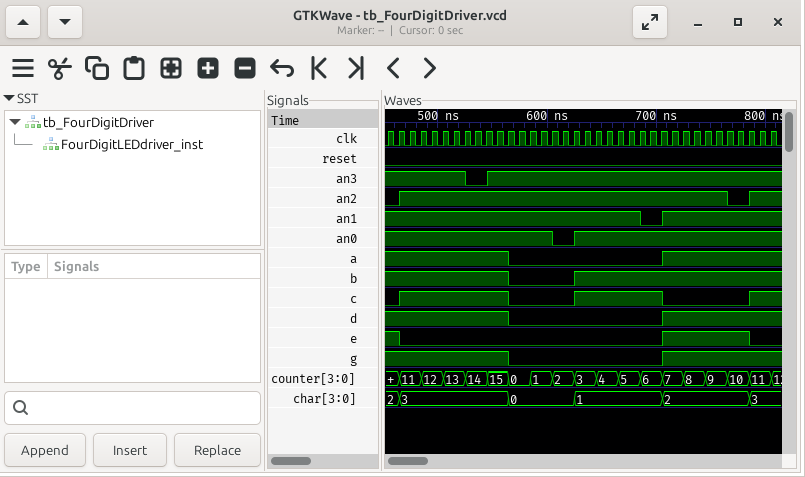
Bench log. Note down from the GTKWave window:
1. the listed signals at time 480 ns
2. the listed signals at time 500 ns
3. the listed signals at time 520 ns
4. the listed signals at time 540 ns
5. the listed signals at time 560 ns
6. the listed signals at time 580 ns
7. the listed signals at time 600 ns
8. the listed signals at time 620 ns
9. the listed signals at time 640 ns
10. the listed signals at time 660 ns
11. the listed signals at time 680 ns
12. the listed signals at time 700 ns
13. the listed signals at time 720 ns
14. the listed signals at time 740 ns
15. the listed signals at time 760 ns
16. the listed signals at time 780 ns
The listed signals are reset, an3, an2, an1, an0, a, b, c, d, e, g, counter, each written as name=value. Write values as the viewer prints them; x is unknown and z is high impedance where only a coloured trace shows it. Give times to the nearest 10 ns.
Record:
reset=0, an3=1, an2=1, an1=1, an0=1, a=1, b=1, c=1, d=1, e=0, g=1, counter=11
reset=0, an3=1, an2=1, an1=1, an0=1, a=1, b=1, c=1, d=1, e=0, g=1, counter=12
reset=0, an3=1, an2=1, an1=1, an0=1, a=1, b=1, c=1, d=1, e=0, g=1, counter=13
reset=0, an3=0, an2=1, an1=1, an0=1, a=1, b=1, c=1, d=1, e=0, g=1, counter=14
reset=0, an3=1, an2=1, an1=1, an0=1, a=1, b=1, c=1, d=1, e=0, g=1, counter=15
reset=0, an3=1, an2=1, an1=1, an0=1, a=0, b=0, c=0, d=0, e=0, g=0, counter=0
reset=0, an3=1, an2=1, an1=1, an0=1, a=0, b=0, c=0, d=0, e=0, g=0, counter=1
reset=0, an3=1, an2=1, an1=1, an0=0, a=0, b=0, c=0, d=0, e=0, g=0, counter=2
reset=0, an3=1, an2=1, an1=1, an0=1, a=0, b=1, c=1, d=0, e=0, g=0, counter=3
reset=0, an3=1, an2=1, an1=1, an0=1, a=0, b=1, c=1, d=0, e=0, g=0, counter=4
reset=0, an3=1, an2=1, an1=1, an0=1, a=0, b=1, c=1, d=0, e=0, g=0, counter=5
reset=0, an3=1, an2=1, an1=0, an0=1, a=0, b=1, c=1, d=0, e=0, g=0, counter=6
reset=0, an3=1, an2=1, an1=1, an0=1, a=1, b=1, c=0, d=1, e=1, g=1, counter=7
reset=0, an3=1, an2=1, an1=1, an0=1, a=1, b=1, c=0, d=1, e=1, g=1, counter=8
reset=0, an3=1, an2=1, an1=1, an0=1, a=1, b=1, c=0, d=1, e=1, g=1, counter=9
reset=0, an3=1, an2=0, an1=1, an0=1, a=1, b=1, c=0, d=1, e=1, g=1, counter=10
